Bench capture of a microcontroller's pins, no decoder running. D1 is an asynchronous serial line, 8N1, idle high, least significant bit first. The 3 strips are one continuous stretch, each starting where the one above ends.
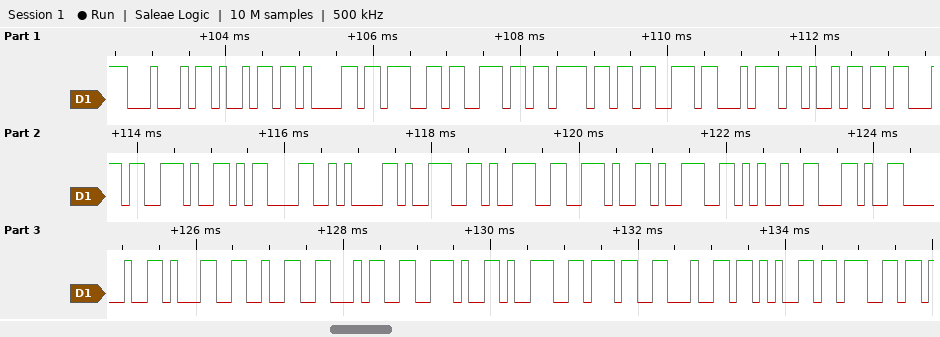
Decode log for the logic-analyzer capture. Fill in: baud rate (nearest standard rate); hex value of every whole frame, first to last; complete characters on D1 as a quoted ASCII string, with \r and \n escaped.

9600 baud
0x44 0x69 0x61 0x67 0x6E 0x6F 0x73 0x74 0x69 0x63 0x2E 0x0D 0x0A 0x39 0x39 0x2E 0x39 0x25 0x2C 0x20 0x31 0x32 0x34 0x2E 0x39 0x37 0x64 0x65 0x67
"Diagnostic.\r\n99.9%, 124.97deg"
